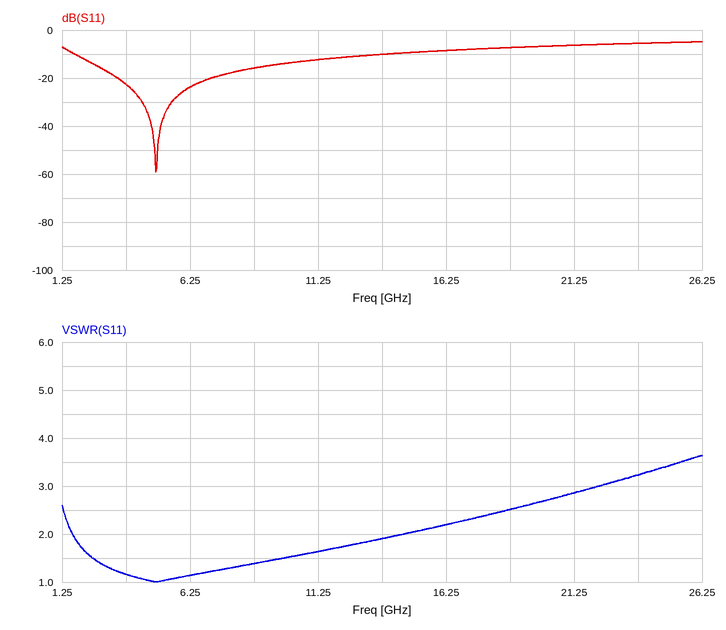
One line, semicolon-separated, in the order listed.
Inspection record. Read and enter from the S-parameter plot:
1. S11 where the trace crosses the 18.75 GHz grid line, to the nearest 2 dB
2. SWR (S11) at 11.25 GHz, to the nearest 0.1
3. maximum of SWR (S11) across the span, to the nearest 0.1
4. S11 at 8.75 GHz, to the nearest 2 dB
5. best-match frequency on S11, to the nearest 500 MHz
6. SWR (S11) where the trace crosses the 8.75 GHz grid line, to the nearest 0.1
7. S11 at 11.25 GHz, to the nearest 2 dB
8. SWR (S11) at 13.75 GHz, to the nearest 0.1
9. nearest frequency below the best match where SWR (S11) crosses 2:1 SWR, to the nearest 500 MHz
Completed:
-8 dB; 1.6; 3.6; -16 dB; 5.0 GHz; 1.4; -12 dB; 1.9; 1.5 GHz
